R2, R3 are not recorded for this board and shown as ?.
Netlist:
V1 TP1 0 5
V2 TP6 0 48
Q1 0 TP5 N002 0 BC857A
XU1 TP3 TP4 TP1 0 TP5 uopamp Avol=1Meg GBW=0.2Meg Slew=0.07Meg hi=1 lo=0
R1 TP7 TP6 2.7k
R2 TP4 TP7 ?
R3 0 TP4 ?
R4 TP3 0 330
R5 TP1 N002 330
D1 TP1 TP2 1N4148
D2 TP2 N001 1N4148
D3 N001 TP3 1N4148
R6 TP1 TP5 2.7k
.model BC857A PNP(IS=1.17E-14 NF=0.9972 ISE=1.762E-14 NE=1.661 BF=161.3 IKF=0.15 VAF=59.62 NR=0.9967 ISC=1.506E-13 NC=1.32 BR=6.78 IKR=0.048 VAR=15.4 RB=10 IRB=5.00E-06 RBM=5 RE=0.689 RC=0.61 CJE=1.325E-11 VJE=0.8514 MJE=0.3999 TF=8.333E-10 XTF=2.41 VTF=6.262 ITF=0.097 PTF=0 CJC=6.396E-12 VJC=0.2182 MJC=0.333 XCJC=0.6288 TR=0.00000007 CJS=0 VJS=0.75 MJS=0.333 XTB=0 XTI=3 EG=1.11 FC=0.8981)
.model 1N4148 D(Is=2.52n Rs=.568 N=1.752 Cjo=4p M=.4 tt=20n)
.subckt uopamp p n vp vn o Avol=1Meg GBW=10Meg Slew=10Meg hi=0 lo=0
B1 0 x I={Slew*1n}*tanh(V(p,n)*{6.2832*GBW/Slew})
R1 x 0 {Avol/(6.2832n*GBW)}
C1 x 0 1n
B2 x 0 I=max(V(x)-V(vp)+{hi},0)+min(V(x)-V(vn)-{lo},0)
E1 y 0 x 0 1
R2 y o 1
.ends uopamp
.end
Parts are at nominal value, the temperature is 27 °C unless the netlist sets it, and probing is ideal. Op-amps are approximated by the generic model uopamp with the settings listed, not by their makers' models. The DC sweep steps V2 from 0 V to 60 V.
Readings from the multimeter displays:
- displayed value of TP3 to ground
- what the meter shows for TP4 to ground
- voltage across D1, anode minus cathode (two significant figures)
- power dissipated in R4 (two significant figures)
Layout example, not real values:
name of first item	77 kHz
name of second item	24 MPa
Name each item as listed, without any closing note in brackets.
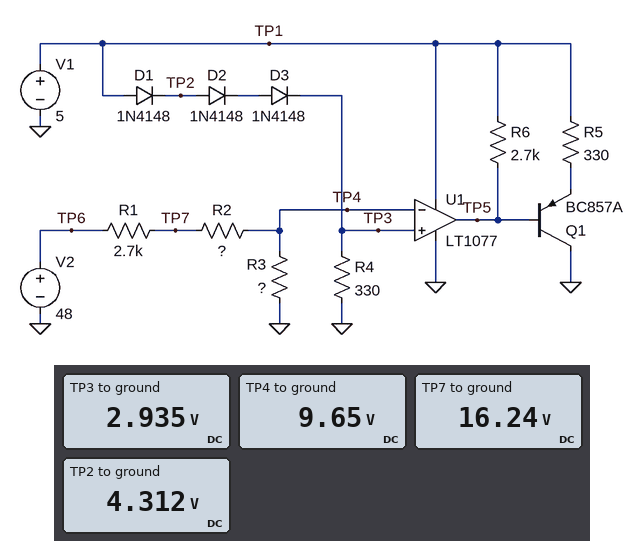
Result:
displayed value of TP3 to ground	2.935 V
what the meter shows for TP4 to ground	9.65 V
voltage across D1, anode minus cathode	690 mV
power dissipated in R4	26 mW
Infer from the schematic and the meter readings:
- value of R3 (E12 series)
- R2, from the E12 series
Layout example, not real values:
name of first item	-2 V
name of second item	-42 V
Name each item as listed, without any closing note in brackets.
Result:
value of R3	820 Ω
R2, from the E12 series	560 Ω
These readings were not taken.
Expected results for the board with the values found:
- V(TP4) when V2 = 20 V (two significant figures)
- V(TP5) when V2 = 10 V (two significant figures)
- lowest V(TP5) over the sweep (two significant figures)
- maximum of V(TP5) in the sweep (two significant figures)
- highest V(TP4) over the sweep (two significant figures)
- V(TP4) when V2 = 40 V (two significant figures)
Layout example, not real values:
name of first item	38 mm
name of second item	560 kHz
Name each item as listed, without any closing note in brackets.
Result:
V(TP4) when V2 = 20 V	4.0 V
V(TP5) when V2 = 10 V	4.0 V
lowest V(TP5) over the sweep	1.9 mV
maximum of V(TP5) in the sweep	4.0 V
highest V(TP4) over the sweep	12 V
V(TP4) when V2 = 40 V	8.0 V
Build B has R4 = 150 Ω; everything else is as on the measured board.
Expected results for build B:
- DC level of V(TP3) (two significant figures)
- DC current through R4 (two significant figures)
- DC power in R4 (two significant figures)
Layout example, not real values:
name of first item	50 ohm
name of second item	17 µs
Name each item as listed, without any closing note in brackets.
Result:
DC level of V(TP3)	2.8 V
DC current through R4	19 mA
DC power in R4	53 mW
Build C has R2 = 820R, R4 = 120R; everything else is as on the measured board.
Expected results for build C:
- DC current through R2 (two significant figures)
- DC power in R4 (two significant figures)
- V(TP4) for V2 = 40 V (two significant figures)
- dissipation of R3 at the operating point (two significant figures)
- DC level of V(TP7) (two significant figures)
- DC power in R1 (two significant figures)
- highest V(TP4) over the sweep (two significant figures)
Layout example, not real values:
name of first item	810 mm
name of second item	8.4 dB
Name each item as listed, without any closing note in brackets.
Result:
DC current through R2	11 mA
DC power in R4	64 mW
V(TP4) for V2 = 40 V	7.6 V
dissipation of R3 at the operating point	100 mW
DC level of V(TP7)	18 V
DC power in R1	330 mW
highest V(TP4) over the sweep	11 V
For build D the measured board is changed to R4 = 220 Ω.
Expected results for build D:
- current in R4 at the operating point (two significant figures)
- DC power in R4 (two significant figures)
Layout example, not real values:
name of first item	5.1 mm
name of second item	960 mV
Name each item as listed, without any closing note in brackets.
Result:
current in R4 at the operating point	13 mA
DC power in R4	38 mW
